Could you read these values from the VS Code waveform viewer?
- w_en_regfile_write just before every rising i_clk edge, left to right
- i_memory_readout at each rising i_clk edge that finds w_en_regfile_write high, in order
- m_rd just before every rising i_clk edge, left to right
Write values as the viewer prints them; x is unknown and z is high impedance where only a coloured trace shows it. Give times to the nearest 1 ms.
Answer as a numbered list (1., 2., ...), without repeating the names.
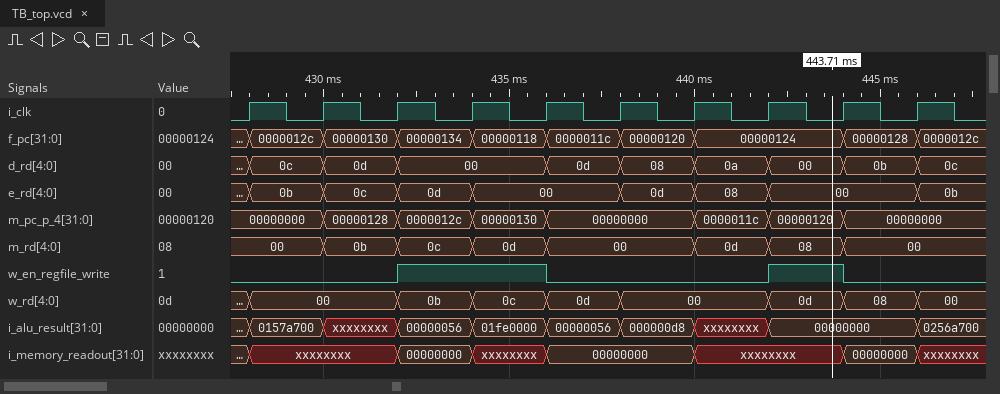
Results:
1. 0 0 0 1 1 0 0 0 1 0
2. 00000000, xxxxxxxx, xxxxxxxx
3. 00, 00, 0b, 0c, 0d, 00, 00, 0d, 08, 00
